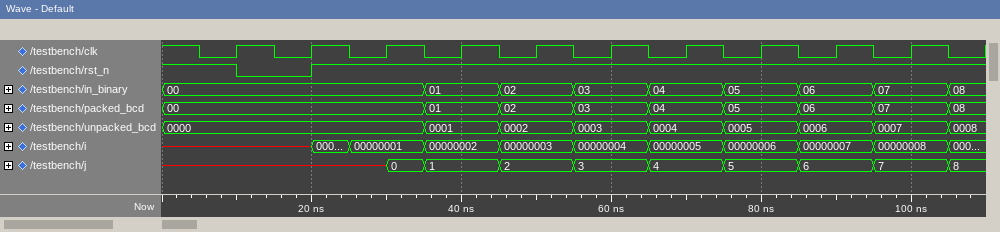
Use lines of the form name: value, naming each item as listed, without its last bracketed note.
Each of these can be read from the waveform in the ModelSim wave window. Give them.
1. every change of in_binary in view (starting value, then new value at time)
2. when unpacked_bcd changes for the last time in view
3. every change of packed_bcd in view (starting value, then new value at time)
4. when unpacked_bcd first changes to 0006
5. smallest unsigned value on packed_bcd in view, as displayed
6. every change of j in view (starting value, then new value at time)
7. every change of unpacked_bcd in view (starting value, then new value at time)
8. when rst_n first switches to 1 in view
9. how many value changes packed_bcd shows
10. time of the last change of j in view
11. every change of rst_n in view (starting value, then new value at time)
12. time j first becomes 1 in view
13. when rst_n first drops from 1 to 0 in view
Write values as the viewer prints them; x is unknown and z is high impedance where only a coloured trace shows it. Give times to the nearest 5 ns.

every change of in_binary in view: 00, 01 at 35 ns, 02 at 45 ns, 03 at 55 ns, 04 at 65 ns, 05 at 75 ns, 06 at 85 ns, 07 at 95 ns, 08 at 105 ns
when unpacked_bcd changes for the last time in view: 105 ns
every change of packed_bcd in view: 00, 01 at 35 ns, 02 at 45 ns, 03 at 55 ns, 04 at 65 ns, 05 at 75 ns, 06 at 85 ns, 07 at 95 ns, 08 at 105 ns
when unpacked_bcd first changes to 0006: 85 ns
smallest unsigned value on packed_bcd in view, as displayed: 00
every change of j in view: x, 0 at 30 ns, 1 at 35 ns, 2 at 45 ns, 3 at 55 ns, 4 at 65 ns, 5 at 75 ns, 6 at 85 ns, 7 at 95 ns, 8 at 105 ns
every change of unpacked_bcd in view: 0000, 0001 at 35 ns, 0002 at 45 ns, 0003 at 55 ns, 0004 at 65 ns, 0005 at 75 ns, 0006 at 85 ns, 0007 at 95 ns, 0008 at 105 ns
when rst_n first switches to 1 in view: 20 ns
how many value changes packed_bcd shows: 8
time of the last change of j in view: 105 ns
every change of rst_n in view: 1, 0 at 10 ns, 1 at 20 ns
time j first becomes 1 in view: 35 ns
when rst_n first drops from 1 to 0 in view: 10 ns
